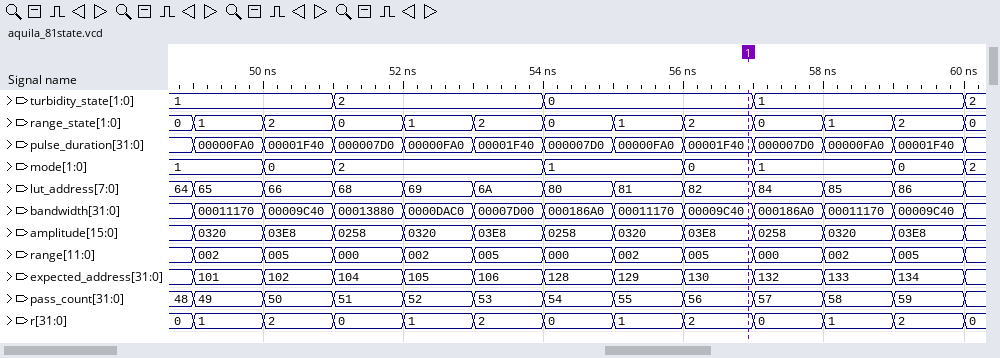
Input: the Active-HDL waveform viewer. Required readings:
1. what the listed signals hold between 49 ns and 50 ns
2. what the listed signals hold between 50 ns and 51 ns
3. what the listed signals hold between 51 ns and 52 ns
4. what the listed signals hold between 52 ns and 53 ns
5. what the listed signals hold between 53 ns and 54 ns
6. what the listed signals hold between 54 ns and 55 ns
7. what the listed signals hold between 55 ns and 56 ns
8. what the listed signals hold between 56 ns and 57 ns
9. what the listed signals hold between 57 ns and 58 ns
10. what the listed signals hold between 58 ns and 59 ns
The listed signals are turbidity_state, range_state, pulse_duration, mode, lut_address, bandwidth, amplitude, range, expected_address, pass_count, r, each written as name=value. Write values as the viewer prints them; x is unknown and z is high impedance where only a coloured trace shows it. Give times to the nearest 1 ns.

turbidity_state=1, range_state=1, pulse_duration=00000FA0, mode=1, lut_address=65, bandwidth=00011170, amplitude=0320, range=002, expected_address=101, pass_count=49, r=1
turbidity_state=1, range_state=2, pulse_duration=00001F40, mode=0, lut_address=66, bandwidth=00009C40, amplitude=03E8, range=005, expected_address=102, pass_count=50, r=2
turbidity_state=2, range_state=0, pulse_duration=000007D0, mode=2, lut_address=68, bandwidth=00013880, amplitude=0258, range=000, expected_address=104, pass_count=51, r=0
turbidity_state=2, range_state=1, pulse_duration=00000FA0, mode=2, lut_address=69, bandwidth=0000DAC0, amplitude=0320, range=002, expected_address=105, pass_count=52, r=1
turbidity_state=2, range_state=2, pulse_duration=00001F40, mode=2, lut_address=6A, bandwidth=00007D00, amplitude=03E8, range=005, expected_address=106, pass_count=53, r=2
turbidity_state=0, range_state=0, pulse_duration=000007D0, mode=1, lut_address=80, bandwidth=000186A0, amplitude=0258, range=000, expected_address=128, pass_count=54, r=0
turbidity_state=0, range_state=1, pulse_duration=00000FA0, mode=1, lut_address=81, bandwidth=00011170, amplitude=0320, range=002, expected_address=129, pass_count=55, r=1
turbidity_state=0, range_state=2, pulse_duration=00001F40, mode=0, lut_address=82, bandwidth=00009C40, amplitude=03E8, range=005, expected_address=130, pass_count=56, r=2
turbidity_state=1, range_state=0, pulse_duration=000007D0, mode=1, lut_address=84, bandwidth=000186A0, amplitude=0258, range=000, expected_address=132, pass_count=57, r=0
turbidity_state=1, range_state=1, pulse_duration=00000FA0, mode=1, lut_address=85, bandwidth=00011170, amplitude=0320, range=002, expected_address=133, pass_count=58, r=1
